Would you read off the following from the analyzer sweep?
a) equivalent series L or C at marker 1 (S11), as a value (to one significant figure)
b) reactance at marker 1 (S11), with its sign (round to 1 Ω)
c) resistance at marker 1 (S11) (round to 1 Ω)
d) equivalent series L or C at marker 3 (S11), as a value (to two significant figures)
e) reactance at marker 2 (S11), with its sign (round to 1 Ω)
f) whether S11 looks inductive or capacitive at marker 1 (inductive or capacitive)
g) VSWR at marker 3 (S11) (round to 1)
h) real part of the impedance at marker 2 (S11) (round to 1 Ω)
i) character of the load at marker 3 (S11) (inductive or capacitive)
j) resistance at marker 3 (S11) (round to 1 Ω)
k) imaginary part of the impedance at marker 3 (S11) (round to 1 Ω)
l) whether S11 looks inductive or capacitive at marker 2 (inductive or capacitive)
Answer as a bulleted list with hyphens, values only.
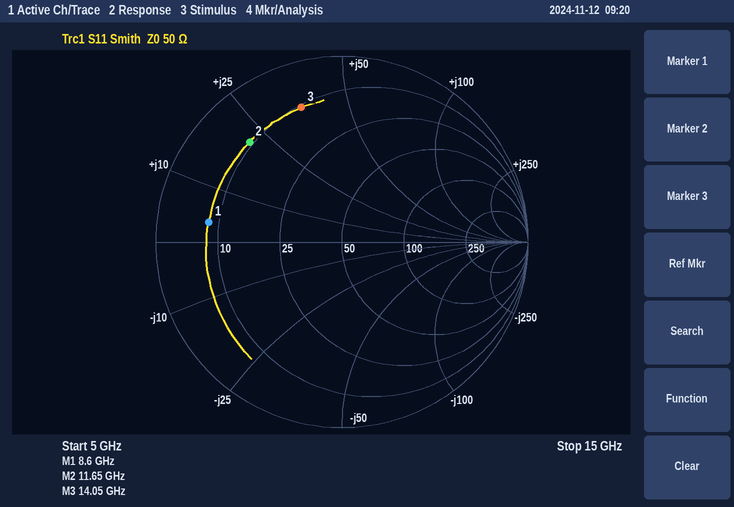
- 70 pH
- +4 Ω
- 8 Ω
- 410 pH
- +21 Ω
- inductive
- 7
- 9 Ω
- inductive
- 11 Ω
- +36 Ω
- inductive
